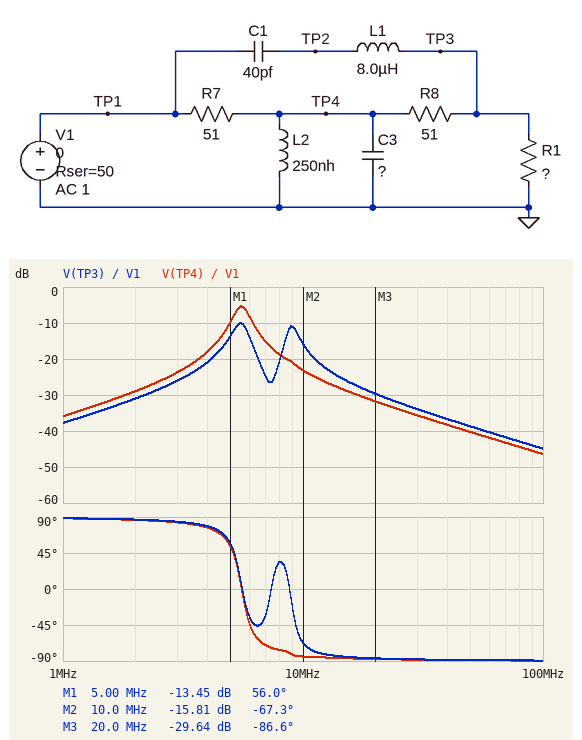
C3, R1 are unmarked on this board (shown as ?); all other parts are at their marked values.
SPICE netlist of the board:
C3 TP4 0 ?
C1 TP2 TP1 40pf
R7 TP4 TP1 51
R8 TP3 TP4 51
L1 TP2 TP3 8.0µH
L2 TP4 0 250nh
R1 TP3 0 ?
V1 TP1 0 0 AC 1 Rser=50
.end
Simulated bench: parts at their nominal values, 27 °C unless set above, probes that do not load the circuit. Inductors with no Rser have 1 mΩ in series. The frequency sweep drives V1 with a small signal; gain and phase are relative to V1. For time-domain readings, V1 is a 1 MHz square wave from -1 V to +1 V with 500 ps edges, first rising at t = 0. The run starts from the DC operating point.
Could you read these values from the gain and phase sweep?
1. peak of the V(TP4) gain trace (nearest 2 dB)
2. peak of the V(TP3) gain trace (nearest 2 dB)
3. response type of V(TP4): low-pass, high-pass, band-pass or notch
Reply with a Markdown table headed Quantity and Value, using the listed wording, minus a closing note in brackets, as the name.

| Quantity | Value |
|---|---|
| peak of the V(TP4) gain trace | -6 dB |
| peak of the V(TP3) gain trace | -10 dB |
| response type of V(TP4): low-pass, high-pass, band-pass or notch | band-pass |
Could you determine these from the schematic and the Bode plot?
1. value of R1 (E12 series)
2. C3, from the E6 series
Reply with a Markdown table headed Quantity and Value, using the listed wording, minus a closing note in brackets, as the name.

| Quantity | Value |
|---|---|
| value of R1 | 68 Ω |
| C3, from the E6 series | 3.3 nF |
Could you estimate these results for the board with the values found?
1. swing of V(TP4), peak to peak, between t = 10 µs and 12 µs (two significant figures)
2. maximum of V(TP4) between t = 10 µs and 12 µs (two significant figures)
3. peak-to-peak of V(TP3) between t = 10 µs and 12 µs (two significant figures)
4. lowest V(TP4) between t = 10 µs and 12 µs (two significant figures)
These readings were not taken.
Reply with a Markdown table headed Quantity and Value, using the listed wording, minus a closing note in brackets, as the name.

| Quantity | Value |
|---|---|
| swing of V(TP4), peak to peak, between t = 10 µs and 12 µs | 300 mV |
| maximum of V(TP4) between t = 10 µs and 12 µs | 150 mV |
| peak-to-peak of V(TP3) between t = 10 µs and 12 µs | 310 mV |
| lowest V(TP4) between t = 10 µs and 12 µs | -150 mV |
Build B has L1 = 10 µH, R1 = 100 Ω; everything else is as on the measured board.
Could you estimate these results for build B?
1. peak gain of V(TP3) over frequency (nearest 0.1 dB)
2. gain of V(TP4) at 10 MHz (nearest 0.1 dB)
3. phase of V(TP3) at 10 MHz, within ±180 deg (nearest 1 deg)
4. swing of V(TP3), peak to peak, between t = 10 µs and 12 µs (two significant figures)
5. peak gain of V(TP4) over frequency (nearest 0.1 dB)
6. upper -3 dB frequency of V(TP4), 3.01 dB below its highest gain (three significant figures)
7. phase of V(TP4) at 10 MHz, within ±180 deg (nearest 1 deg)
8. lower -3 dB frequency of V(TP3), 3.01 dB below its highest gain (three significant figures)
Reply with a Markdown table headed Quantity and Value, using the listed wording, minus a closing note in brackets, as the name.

| Quantity | Value |
|---|---|
| peak gain of V(TP3) over frequency | -7.8 dB |
| gain of V(TP4) at 10 MHz | -23.2 dB |
| phase of V(TP3) at 10 MHz, within ±180 deg | -79 deg |
| swing of V(TP3), peak to peak, between t = 10 µs and 12 µs | 300 mV |
| peak gain of V(TP4) over frequency | -4.4 dB |
| upper -3 dB frequency of V(TP4), 3.01 dB below its highest gain | 5.95 MHz |
| phase of V(TP4) at 10 MHz, within ±180 deg | -85 deg |
| lower -3 dB frequency of V(TP3), 3.01 dB below its highest gain | 5.09 MHz |
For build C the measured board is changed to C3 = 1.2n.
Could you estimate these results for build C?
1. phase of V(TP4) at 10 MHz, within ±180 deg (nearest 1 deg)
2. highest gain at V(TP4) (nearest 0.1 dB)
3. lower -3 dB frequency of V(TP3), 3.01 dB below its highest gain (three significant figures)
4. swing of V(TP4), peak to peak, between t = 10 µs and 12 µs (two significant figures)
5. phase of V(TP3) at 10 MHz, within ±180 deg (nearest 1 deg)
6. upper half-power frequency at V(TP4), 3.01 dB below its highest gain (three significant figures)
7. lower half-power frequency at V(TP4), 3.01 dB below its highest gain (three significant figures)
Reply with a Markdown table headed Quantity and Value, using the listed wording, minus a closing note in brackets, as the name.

| Quantity | Value |
|---|---|
| phase of V(TP4) at 10 MHz, within ±180 deg | -34 deg |
| highest gain at V(TP4) | -4.9 dB |
| lower -3 dB frequency of V(TP3), 3.01 dB below its highest gain | 8.22 MHz |
| swing of V(TP4), peak to peak, between t = 10 µs and 12 µs | 490 mV |
| phase of V(TP3) at 10 MHz, within ±180 deg | -42 deg |
| upper half-power frequency at V(TP4), 3.01 dB below its highest gain | 10.4 MHz |
| lower half-power frequency at V(TP4), 3.01 dB below its highest gain | 8.12 MHz |
